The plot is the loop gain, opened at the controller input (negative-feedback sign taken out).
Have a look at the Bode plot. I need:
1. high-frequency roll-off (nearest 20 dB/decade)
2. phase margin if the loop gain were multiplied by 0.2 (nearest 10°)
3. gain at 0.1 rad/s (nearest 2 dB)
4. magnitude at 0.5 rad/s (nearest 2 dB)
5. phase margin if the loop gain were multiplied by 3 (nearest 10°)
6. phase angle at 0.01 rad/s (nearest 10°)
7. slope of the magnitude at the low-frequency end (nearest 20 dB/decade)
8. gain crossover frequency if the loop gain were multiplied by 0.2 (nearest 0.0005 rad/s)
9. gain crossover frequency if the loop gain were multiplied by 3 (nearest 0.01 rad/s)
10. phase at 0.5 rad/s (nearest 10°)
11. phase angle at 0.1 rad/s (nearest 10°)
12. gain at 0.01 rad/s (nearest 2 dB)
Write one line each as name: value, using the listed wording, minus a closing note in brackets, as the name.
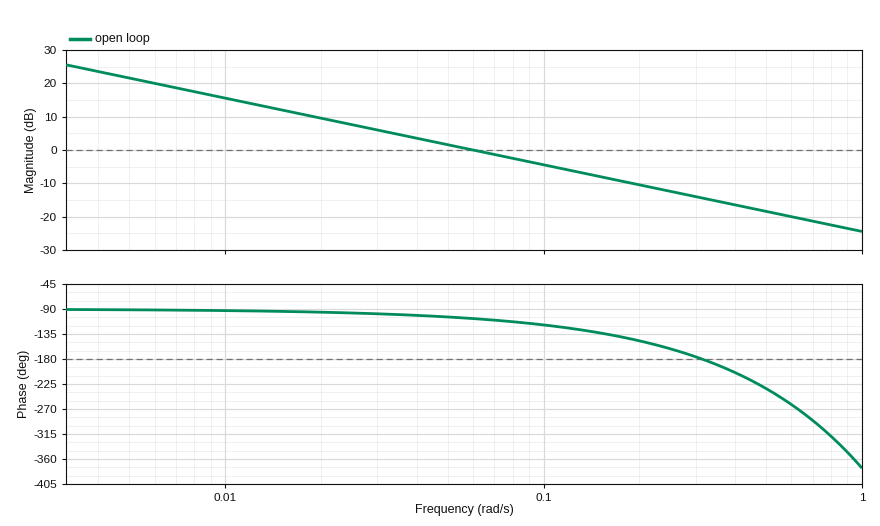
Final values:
high-frequency roll-off: -20 dB/decade
phase margin if the loop gain were multiplied by 0.2: 90°
gain at 0.1 rad/s: -4 dB
magnitude at 0.5 rad/s: -18 dB
phase margin if the loop gain were multiplied by 3: 40°
phase angle at 0.01 rad/s: -90°
slope of the magnitude at the low-frequency end: -20 dB/decade
gain crossover frequency if the loop gain were multiplied by 0.2: 0.0120 rad/s
gain crossover frequency if the loop gain were multiplied by 3: 0.18 rad/s
phase at 0.5 rad/s: -230°
phase angle at 0.1 rad/s: -120°
gain at 0.01 rad/s: 16 dB
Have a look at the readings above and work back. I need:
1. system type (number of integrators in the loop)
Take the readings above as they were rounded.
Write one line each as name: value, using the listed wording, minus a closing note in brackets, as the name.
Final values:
system type: 1
